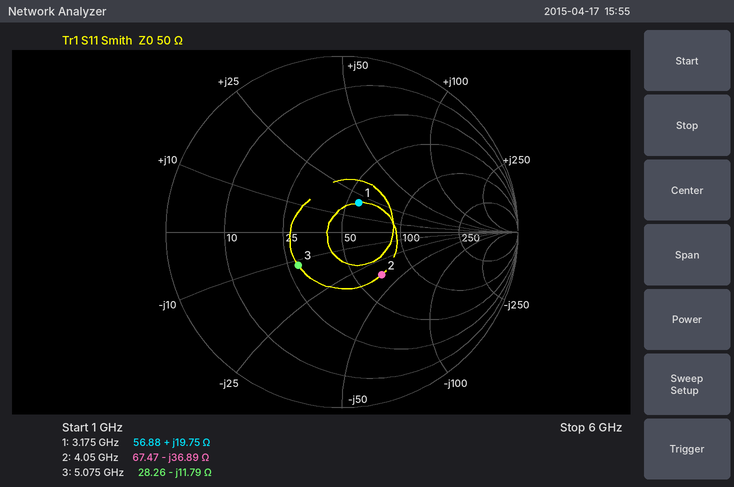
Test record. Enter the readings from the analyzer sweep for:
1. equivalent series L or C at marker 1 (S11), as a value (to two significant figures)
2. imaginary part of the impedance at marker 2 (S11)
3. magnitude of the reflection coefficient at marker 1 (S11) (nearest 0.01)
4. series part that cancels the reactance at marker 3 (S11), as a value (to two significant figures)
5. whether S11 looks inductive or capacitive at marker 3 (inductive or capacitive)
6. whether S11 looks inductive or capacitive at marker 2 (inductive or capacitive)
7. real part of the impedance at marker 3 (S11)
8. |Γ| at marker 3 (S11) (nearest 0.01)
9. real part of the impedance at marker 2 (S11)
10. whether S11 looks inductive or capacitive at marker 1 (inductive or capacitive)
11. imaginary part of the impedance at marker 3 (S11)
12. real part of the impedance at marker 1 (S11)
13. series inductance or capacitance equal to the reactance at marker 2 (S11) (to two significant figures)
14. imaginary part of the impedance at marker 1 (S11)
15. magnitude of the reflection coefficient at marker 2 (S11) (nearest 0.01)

990 pH
-36.89 Ω
0.19
370 pH
capacitive
capacitive
28.26 Ω
0.31
67.47 Ω
inductive
-11.79 Ω
56.88 Ω
1.1 pF
+19.75 Ω
0.33
